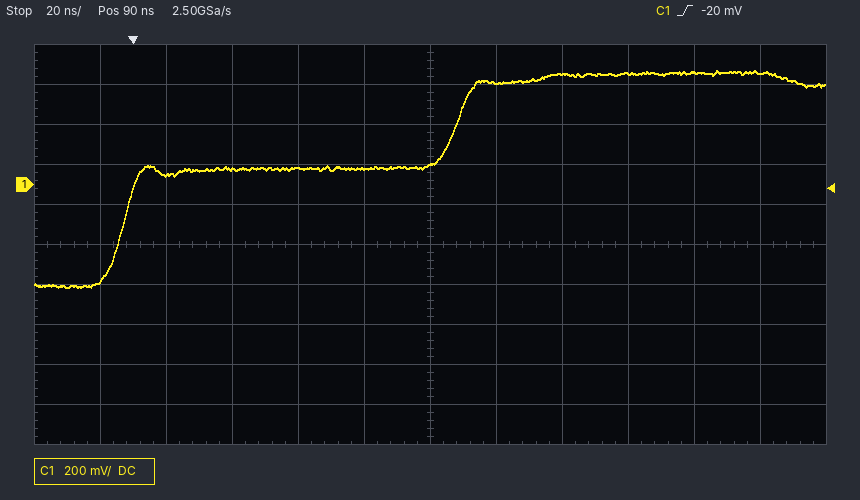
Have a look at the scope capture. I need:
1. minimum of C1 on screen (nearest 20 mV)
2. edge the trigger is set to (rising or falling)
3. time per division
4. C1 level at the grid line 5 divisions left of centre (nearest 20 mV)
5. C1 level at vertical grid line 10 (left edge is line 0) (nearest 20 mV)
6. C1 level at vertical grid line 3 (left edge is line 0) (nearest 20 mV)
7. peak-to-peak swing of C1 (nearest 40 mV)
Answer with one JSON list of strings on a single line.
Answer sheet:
["-520 mV", "rising", "20 ns", "-480 mV", "560 mV", "80 mV", "1.08 V"]
